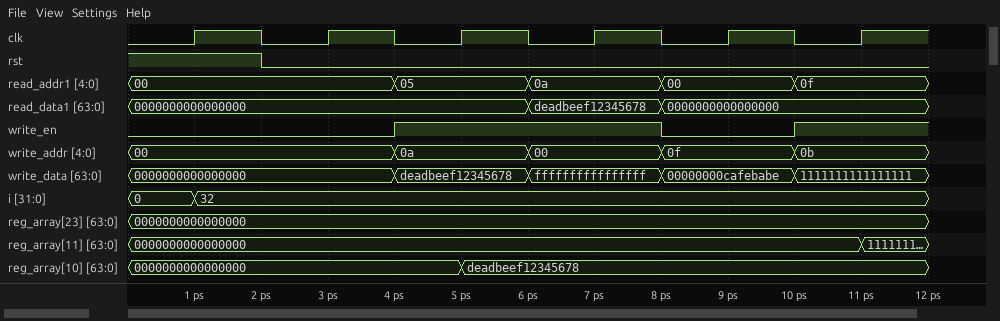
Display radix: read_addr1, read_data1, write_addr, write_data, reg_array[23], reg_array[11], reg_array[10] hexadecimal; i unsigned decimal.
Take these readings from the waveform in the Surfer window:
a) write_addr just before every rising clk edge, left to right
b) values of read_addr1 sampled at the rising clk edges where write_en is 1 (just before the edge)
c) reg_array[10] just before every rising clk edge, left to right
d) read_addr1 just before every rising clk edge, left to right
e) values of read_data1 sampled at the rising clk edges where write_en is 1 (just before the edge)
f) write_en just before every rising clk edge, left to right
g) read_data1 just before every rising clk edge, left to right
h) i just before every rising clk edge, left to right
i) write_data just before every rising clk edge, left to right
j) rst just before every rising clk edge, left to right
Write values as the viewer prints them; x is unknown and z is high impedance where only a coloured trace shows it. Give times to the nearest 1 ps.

00, 00, 0a, 00, 0f, 0b
05, 0a, 0f
0000000000000000, 0000000000000000, 0000000000000000, deadbeef12345678, deadbeef12345678, deadbeef12345678
00, 00, 05, 0a, 00, 0f
0000000000000000, deadbeef12345678, 0000000000000000
0 0 1 1 0 1
0000000000000000, 0000000000000000, 0000000000000000, deadbeef12345678, 0000000000000000, 0000000000000000
0, 32, 32, 32, 32, 32
0000000000000000, 0000000000000000, deadbeef12345678, ffffffffffffffff, 00000000cafebabe, 1111111111111111
1 0 0 0 0 0
